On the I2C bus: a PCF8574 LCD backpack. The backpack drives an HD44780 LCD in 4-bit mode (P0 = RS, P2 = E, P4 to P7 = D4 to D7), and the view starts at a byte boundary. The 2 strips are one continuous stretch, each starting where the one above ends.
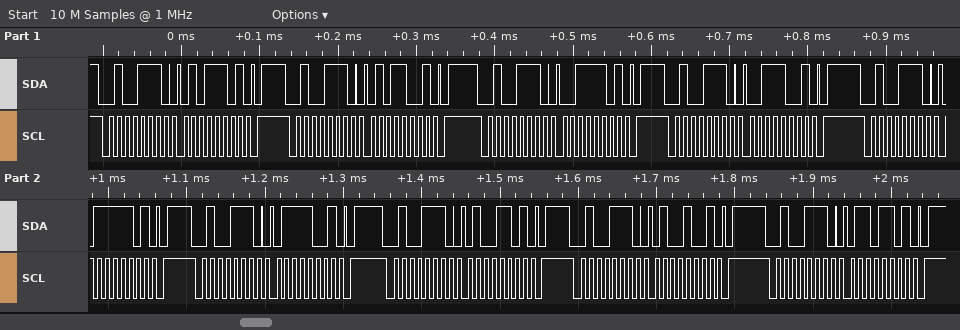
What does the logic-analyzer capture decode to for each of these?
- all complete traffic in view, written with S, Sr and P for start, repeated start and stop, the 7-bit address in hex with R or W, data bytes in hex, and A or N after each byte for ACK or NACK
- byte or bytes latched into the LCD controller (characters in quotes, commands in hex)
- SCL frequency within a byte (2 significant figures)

S 27W A 5D A P S 27W A 59 A P S 27W A 3D A P S 27W A 39 A P S 27W A 7D A P S 27W A 79 A P S 27W A 4D A P S 27W A 49 A P S 27W A 6D A P
'S' 't'
100 kHz
